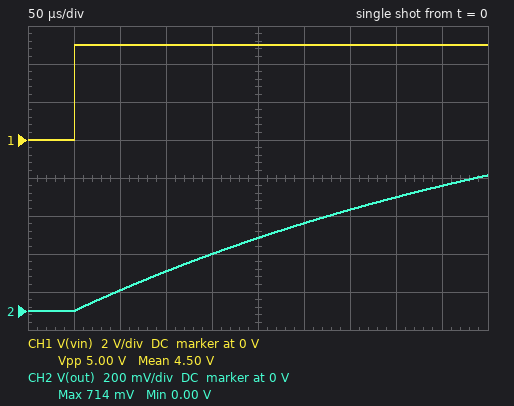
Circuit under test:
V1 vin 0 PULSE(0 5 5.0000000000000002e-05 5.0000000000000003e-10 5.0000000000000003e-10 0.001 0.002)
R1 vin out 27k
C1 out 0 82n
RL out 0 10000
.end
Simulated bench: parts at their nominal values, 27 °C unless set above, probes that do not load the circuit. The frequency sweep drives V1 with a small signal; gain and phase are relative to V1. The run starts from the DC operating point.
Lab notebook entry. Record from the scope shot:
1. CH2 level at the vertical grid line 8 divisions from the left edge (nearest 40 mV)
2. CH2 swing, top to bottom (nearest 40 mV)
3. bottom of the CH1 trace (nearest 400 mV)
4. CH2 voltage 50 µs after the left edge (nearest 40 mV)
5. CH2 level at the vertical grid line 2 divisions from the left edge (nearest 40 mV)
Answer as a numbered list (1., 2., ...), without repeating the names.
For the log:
1. 600 mV
2. 720 mV
3. 0 V
4. 0 V
5. 120 mV
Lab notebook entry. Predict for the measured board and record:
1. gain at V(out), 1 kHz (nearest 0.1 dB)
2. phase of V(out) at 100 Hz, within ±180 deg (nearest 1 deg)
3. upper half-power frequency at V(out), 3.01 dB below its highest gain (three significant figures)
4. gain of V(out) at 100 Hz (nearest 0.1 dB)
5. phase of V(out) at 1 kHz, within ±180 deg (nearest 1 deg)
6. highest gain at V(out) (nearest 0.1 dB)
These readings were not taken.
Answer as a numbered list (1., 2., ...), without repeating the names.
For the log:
1. -23.2 dB
2. -21 deg
3. 266 Hz
4. -11.9 dB
5. -75 deg
6. -11.4 dB
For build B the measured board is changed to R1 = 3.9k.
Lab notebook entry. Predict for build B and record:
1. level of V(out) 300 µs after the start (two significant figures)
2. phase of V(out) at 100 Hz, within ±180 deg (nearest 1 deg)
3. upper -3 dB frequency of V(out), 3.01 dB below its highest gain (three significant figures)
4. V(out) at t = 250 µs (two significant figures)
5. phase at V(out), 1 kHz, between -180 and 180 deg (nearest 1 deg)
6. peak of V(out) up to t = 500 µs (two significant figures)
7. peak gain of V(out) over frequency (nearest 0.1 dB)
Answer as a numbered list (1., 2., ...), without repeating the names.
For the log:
1. 2.4 V
2. -8 deg
3. 692 Hz
4. 2.1 V
5. -55 deg
6. 3.1 V
7. -2.9 dB
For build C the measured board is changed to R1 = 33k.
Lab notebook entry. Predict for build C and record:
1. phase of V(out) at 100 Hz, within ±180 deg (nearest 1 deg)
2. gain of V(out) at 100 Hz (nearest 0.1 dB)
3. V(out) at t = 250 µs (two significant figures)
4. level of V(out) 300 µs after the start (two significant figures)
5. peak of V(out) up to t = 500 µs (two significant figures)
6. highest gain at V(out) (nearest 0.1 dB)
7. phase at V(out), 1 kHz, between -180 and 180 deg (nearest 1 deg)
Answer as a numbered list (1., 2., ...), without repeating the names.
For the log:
1. -22 deg
2. -13.3 dB
3. 320 mV
4. 380 mV
5. 590 mV
6. -12.7 dB
7. -76 deg
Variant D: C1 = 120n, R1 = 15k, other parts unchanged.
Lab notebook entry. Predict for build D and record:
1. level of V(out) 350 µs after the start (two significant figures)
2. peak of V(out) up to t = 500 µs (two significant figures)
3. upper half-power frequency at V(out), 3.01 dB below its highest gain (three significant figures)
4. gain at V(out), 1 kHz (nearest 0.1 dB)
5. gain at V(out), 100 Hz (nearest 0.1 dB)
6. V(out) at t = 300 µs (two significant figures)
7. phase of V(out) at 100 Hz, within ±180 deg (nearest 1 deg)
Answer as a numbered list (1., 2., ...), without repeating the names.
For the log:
1. 680 mV
2. 930 mV
3. 221 Hz
4. -21.3 dB
5. -8.8 dB
6. 590 mV
7. -24 deg
